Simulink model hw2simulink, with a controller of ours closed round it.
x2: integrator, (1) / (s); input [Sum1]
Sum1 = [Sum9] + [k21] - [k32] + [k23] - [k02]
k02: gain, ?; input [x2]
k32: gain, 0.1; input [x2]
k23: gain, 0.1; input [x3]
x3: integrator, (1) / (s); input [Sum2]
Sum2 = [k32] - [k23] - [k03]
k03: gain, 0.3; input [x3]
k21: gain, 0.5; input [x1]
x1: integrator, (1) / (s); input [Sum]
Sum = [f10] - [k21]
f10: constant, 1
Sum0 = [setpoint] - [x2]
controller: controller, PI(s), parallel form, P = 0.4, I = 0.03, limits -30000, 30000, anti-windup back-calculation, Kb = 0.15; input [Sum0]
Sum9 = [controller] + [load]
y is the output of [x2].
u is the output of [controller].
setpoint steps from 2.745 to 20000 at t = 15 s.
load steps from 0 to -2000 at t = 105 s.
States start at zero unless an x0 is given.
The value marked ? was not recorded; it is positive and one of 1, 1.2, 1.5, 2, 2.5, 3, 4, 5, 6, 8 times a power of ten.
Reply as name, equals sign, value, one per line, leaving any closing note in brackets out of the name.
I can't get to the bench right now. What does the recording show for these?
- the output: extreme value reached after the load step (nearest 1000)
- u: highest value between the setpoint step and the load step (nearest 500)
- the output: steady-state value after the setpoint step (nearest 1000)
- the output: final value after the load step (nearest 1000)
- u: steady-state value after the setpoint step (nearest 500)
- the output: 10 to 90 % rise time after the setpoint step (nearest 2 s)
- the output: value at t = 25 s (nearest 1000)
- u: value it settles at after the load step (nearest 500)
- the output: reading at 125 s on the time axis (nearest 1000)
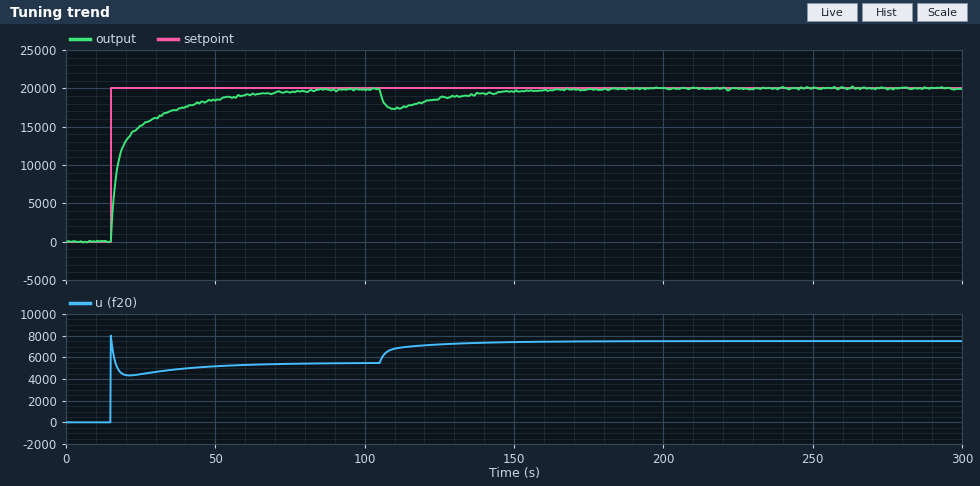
the output: extreme value reached after the load step = 17000
u: highest value between the setpoint step and the load step = 8000
the output: steady-state value after the setpoint step = 20000
the output: final value after the load step = 20000
u: steady-state value after the setpoint step = 5500
the output: 10 to 90 % rise time after the setpoint step = 28 s
the output: value at t = 25 s = 15000
u: value it settles at after the load step = 7500
the output: reading at 125 s on the time axis = 19000
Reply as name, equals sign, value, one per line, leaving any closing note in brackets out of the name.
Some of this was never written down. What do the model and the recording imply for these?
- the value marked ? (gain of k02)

the value marked ? = 0.2
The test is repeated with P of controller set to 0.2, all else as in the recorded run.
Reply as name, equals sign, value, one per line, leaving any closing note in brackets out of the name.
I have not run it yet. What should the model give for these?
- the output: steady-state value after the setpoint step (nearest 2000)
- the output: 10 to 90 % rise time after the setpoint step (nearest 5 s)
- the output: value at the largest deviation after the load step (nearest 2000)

the output: steady-state value after the setpoint step = 20000
the output: 10 to 90 % rise time after the setpoint step = 25 s
the output: value at the largest deviation after the load step = 16000
